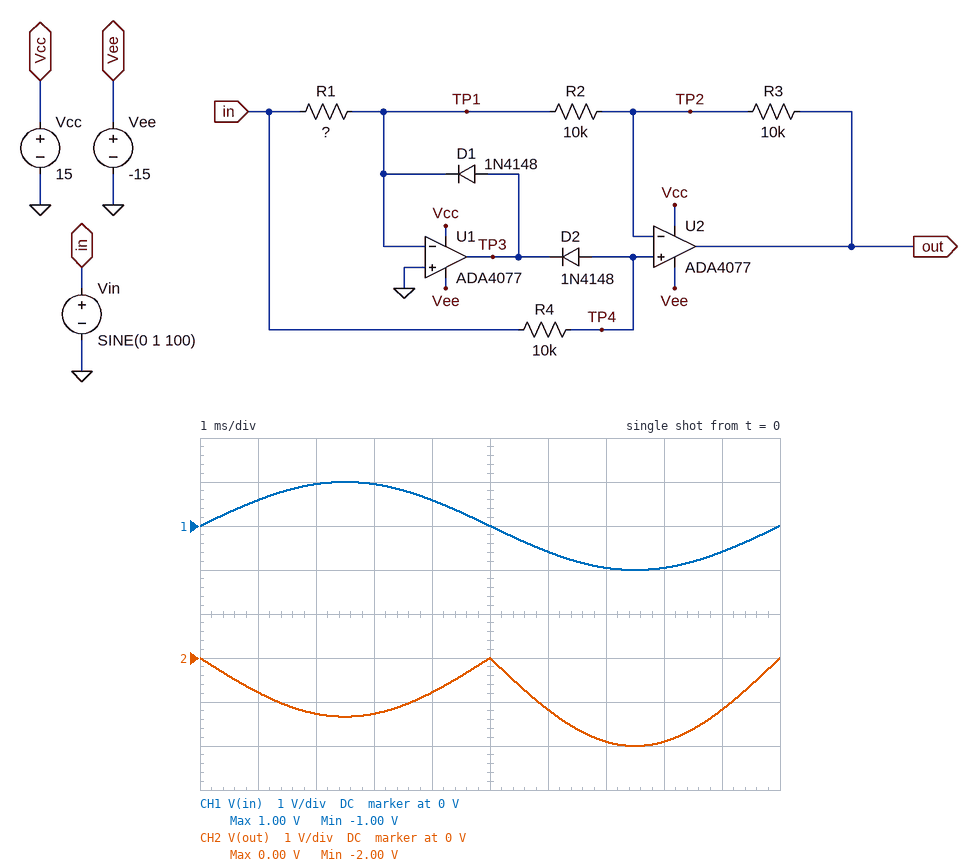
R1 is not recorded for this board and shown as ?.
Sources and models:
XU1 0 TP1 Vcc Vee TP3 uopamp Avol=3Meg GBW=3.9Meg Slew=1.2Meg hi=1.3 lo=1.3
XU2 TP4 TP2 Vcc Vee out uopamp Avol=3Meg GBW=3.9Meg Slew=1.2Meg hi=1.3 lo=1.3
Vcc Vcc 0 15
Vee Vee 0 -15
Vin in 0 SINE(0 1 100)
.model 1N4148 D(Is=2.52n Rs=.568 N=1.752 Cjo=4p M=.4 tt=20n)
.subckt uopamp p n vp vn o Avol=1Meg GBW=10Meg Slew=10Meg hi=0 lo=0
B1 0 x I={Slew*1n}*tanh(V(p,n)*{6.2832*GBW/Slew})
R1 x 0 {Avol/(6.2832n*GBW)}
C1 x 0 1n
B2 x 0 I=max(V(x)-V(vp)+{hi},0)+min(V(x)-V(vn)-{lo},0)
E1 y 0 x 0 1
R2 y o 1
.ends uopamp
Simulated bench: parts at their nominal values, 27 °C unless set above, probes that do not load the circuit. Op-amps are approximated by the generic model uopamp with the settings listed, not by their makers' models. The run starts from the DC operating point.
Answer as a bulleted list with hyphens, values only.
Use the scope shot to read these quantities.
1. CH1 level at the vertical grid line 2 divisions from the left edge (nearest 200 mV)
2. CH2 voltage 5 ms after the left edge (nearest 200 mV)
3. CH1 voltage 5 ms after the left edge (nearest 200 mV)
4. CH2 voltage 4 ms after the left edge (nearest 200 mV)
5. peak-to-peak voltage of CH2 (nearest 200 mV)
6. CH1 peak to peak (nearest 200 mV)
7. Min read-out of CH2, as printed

- 1.0 V
- 0 V
- 0 V
- -800 mV
- 2.0 V
- 2.0 V
- -2.00 V
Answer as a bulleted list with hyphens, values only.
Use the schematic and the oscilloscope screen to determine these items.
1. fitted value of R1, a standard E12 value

- 15 kΩ
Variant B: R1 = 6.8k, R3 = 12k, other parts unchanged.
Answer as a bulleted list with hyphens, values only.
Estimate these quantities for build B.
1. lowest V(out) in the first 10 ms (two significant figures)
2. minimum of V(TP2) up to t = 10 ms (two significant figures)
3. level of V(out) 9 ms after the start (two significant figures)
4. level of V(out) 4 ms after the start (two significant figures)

- -3.2 V
- -1.5 V
- -1.3 V
- -1.9 V
